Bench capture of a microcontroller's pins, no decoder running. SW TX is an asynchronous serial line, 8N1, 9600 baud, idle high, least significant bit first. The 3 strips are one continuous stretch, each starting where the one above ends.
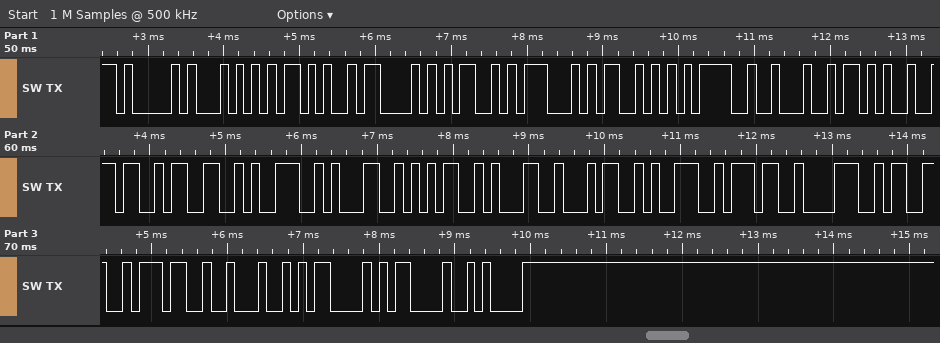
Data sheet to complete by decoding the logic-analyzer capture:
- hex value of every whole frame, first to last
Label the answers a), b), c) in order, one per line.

a) 41 54 2B 43 4D 47 53 3D 22 2B 36 33 39 31 35 31 34 39 37 38 33 37 22 0D 0D 0A
